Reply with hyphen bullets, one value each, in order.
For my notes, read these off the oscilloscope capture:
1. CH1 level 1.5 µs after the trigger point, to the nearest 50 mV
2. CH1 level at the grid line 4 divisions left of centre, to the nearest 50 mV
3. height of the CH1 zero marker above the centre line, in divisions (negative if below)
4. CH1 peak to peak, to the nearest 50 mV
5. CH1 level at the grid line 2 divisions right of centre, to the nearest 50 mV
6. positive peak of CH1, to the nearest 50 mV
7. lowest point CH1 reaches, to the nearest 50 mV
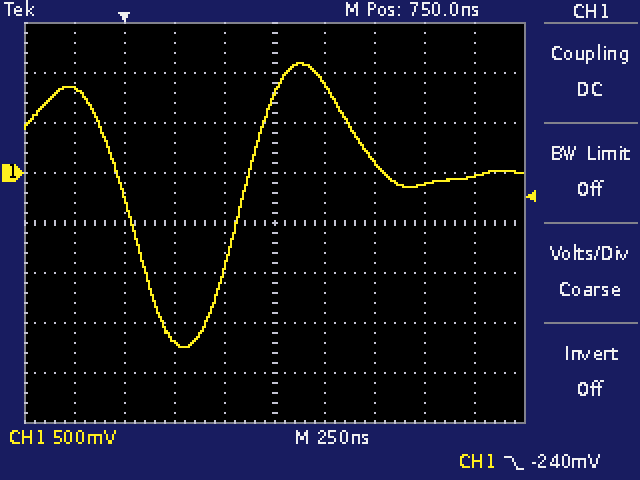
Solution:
- -100 mV
- 850 mV
- +1.0 div
- 2.85 V
- 100 mV
- 1.10 V
- -1.75 V
